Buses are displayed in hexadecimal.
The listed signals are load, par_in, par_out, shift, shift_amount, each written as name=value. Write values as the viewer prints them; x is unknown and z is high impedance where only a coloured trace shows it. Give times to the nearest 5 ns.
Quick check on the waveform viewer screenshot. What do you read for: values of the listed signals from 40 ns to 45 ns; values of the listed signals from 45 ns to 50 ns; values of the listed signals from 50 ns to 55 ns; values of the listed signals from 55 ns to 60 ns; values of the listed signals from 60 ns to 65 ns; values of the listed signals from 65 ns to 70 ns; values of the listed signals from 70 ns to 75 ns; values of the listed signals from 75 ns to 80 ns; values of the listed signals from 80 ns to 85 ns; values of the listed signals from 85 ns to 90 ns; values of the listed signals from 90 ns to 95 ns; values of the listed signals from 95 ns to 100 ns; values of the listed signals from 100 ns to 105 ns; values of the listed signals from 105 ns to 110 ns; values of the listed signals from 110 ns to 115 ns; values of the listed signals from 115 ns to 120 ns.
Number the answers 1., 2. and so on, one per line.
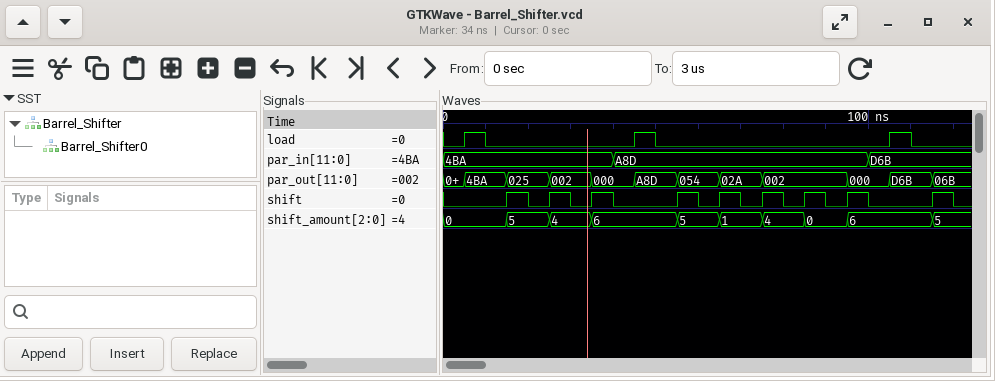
1. load=0, par_in=A8D, par_out=000, shift=0, shift_amount=6
2. load=1, par_in=A8D, par_out=A8D, shift=0, shift_amount=6
3. load=0, par_in=A8D, par_out=A8D, shift=0, shift_amount=6
4. load=0, par_in=A8D, par_out=054, shift=1, shift_amount=5
5. load=0, par_in=A8D, par_out=054, shift=0, shift_amount=5
6. load=0, par_in=A8D, par_out=02A, shift=1, shift_amount=1
7. load=0, par_in=A8D, par_out=02A, shift=0, shift_amount=1
8. load=0, par_in=A8D, par_out=002, shift=1, shift_amount=4
9. load=0, par_in=A8D, par_out=002, shift=0, shift_amount=4
10. load=0, par_in=A8D, par_out=002, shift=1, shift_amount=0
11. load=0, par_in=A8D, par_out=002, shift=0, shift_amount=0
12. load=0, par_in=A8D, par_out=000, shift=1, shift_amount=6
13. load=0, par_in=D6B, par_out=000, shift=0, shift_amount=6
14. load=1, par_in=D6B, par_out=D6B, shift=0, shift_amount=6
15. load=0, par_in=D6B, par_out=D6B, shift=0, shift_amount=6
16. load=0, par_in=D6B, par_out=06B, shift=1, shift_amount=5
